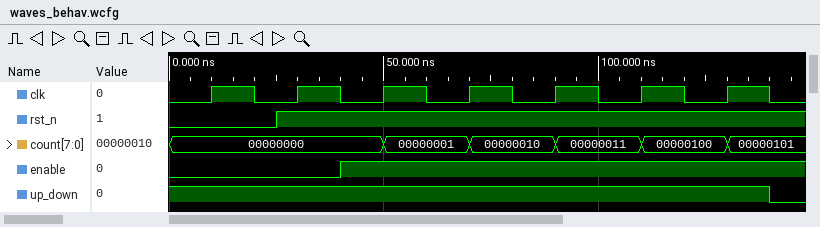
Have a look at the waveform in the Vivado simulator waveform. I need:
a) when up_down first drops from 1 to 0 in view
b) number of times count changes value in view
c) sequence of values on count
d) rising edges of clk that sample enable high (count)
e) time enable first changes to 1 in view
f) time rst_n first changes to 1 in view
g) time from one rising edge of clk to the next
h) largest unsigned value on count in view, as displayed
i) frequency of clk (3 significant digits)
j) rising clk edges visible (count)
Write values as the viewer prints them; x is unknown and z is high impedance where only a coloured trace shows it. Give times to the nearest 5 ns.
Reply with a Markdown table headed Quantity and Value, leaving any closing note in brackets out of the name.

| Quantity | Value |
|---|---|
| when up_down first drops from 1 to 0 in view | 140 ns |
| number of times count changes value in view | 5 |
| sequence of values on count | 00000000, 00000001, 00000010, 00000011, 00000100, 00000101 |
| rising edges of clk that sample enable high | 5 |
| time enable first changes to 1 in view | 40 ns |
| time rst_n first changes to 1 in view | 25 ns |
| time from one rising edge of clk to the next | 20 ns |
| largest unsigned value on count in view, as displayed | 00000101 |
| frequency of clk | 50.0 MHz |
| rising clk edges visible | 7 |
